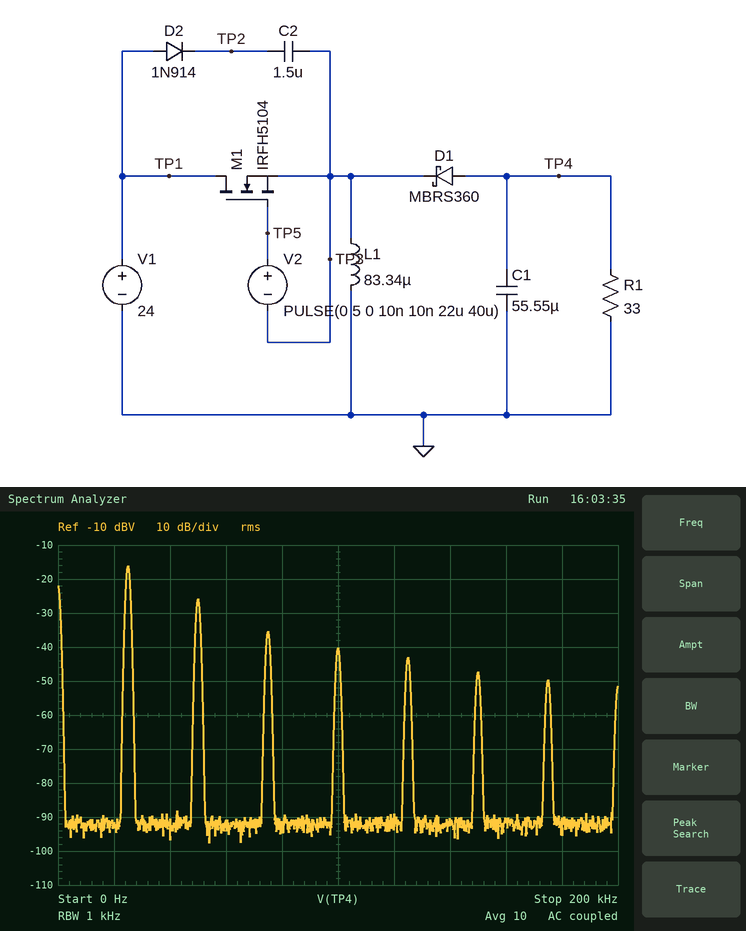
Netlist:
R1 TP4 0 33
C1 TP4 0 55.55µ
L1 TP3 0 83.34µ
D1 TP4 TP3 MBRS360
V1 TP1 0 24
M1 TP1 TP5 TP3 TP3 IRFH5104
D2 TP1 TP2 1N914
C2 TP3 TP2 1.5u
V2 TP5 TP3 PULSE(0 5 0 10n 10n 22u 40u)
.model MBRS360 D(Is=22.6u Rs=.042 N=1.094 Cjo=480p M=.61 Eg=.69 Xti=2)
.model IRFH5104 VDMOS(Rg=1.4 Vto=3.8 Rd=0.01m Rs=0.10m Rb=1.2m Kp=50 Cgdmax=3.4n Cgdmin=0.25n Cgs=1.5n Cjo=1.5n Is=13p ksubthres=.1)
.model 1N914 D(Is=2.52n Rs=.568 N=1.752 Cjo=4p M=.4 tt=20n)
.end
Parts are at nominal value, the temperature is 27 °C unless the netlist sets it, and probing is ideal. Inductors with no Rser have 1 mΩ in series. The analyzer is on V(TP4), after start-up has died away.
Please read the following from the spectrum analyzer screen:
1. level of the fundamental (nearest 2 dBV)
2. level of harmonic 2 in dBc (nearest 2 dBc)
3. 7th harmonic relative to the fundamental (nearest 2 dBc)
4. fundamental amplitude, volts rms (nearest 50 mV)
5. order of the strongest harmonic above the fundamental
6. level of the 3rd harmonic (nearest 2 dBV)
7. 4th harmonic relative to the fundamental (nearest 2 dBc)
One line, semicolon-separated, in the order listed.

-16 dBV; -10 dBc; -34 dBc; 150 mV; 2; -36 dBV; -24 dBc
